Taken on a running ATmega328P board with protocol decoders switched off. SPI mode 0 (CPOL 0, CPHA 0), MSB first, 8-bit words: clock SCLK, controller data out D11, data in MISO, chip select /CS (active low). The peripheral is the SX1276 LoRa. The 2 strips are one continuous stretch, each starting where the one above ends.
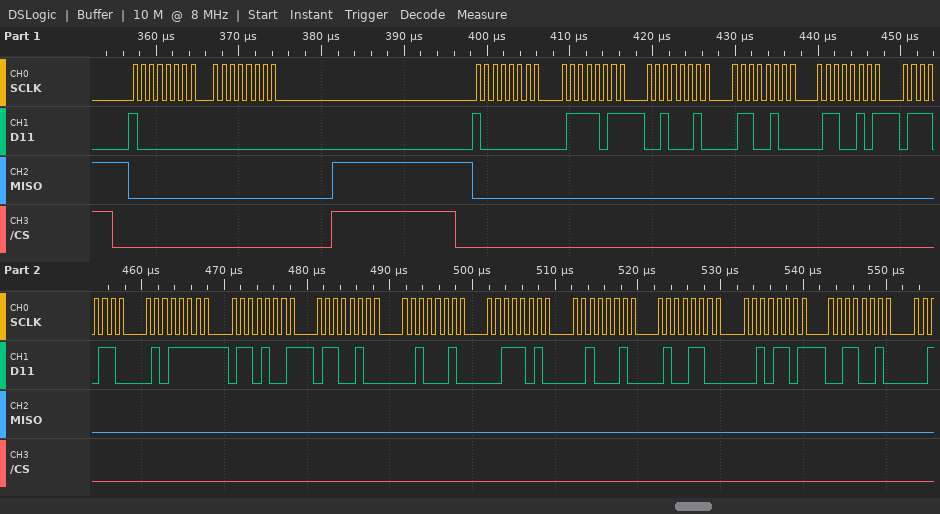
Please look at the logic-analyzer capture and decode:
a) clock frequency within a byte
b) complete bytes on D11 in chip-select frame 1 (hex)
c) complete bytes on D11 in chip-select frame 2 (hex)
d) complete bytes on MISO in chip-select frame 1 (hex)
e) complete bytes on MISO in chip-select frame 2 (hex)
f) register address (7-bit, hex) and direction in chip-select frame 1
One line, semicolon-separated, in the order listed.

1 MHz; 80 00; 80 7B 22 64 65 76 5F 69 64 22 3A 22 4C 2D 32; 00 00; 00 00 00 00 00 00 00 00 00 00 00 00 00 00 00; 0x00 write
